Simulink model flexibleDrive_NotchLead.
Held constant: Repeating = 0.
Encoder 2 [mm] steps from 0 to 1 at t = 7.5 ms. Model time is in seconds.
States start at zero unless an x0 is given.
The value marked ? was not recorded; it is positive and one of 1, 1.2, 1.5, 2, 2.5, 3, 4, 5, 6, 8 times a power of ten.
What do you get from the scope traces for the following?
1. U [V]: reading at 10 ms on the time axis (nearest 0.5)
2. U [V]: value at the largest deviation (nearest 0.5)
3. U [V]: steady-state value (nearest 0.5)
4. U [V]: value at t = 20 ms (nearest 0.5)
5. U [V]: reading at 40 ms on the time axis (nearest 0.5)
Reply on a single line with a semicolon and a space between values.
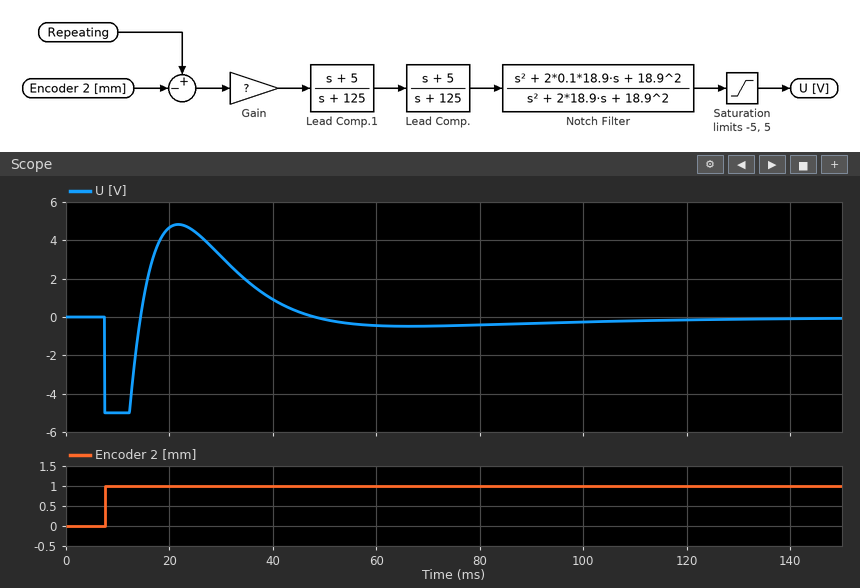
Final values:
-5.0; -5.0; 0.0; 4.5; 1.0
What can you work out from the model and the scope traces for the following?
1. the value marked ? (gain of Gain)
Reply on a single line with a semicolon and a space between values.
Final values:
30
